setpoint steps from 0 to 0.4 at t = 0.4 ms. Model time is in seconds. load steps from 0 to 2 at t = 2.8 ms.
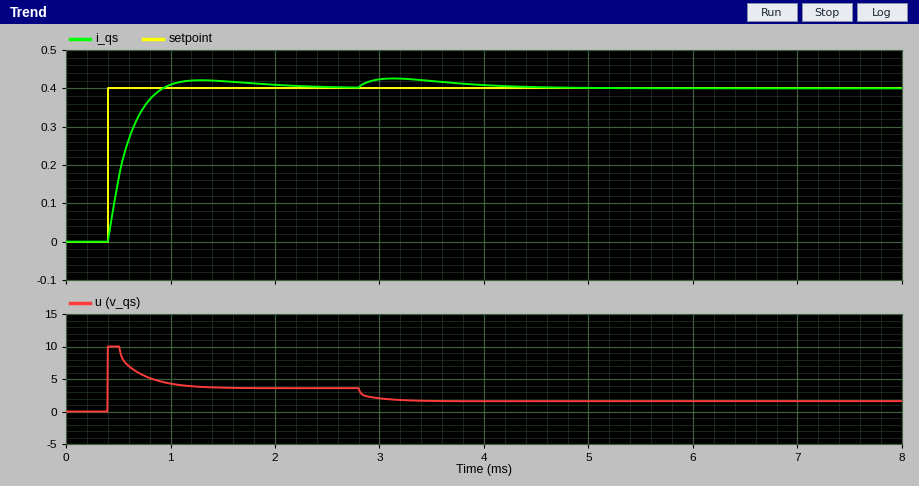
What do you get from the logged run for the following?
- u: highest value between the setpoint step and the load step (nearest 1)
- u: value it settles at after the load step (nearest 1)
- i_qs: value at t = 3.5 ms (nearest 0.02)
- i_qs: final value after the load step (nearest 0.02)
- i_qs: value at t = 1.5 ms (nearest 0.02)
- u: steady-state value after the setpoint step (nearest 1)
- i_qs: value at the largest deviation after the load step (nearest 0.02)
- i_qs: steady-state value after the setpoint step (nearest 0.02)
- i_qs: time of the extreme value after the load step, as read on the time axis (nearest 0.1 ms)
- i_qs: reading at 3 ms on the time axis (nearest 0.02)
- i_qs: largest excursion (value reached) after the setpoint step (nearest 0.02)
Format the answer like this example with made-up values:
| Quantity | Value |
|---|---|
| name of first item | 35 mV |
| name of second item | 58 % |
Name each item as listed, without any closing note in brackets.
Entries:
| Quantity | Value |
|---|---|
| u: highest value between the setpoint step and the load step | 10 |
| u: value it settles at after the load step | 2 |
| i_qs: value at t = 3.5 ms | 0.42 |
| i_qs: final value after the load step | 0.40 |
| i_qs: value at t = 1.5 ms | 0.42 |
| u: steady-state value after the setpoint step | 4 |
| i_qs: value at the largest deviation after the load step | 0.42 |
| i_qs: steady-state value after the setpoint step | 0.40 |
| i_qs: time of the extreme value after the load step, as read on the time axis | 3.1 ms |
| i_qs: reading at 3 ms on the time axis | 0.42 |
| i_qs: largest excursion (value reached) after the setpoint step | 0.42 |
